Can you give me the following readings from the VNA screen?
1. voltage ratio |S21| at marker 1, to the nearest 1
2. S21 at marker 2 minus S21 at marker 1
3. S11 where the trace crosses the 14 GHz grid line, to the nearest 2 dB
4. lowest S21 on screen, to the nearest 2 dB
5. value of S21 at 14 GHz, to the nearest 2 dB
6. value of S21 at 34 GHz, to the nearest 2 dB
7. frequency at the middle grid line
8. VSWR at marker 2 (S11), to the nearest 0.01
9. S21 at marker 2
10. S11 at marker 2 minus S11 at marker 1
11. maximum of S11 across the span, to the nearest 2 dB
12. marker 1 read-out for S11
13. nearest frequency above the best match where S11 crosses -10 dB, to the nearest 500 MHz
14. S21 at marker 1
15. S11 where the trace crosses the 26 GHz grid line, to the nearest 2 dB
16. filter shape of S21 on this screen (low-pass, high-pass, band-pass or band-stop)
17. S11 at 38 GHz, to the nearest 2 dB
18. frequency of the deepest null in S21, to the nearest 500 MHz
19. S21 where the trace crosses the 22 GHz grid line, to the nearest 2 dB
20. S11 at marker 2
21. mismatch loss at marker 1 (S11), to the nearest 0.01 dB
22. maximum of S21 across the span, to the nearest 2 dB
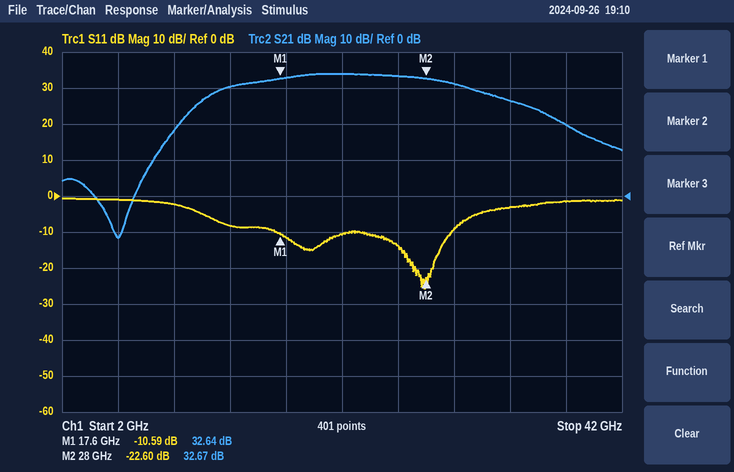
43
0.03 dB
-8 dB
-12 dB
30 dB
26 dB
22 GHz
1.16
32.67 dB
-12.01 dB
0 dB
-10.59 dB
30.0 GHz
32.64 dB
-14 dB
band-pass
-2 dB
6.0 GHz
34 dB
-22.60 dB
0.40 dB
34 dB
